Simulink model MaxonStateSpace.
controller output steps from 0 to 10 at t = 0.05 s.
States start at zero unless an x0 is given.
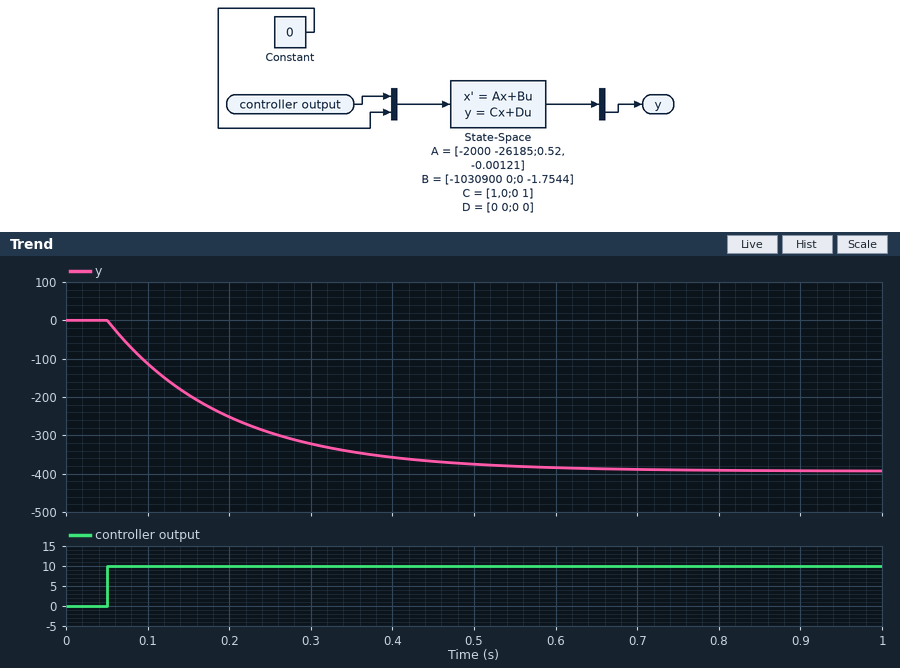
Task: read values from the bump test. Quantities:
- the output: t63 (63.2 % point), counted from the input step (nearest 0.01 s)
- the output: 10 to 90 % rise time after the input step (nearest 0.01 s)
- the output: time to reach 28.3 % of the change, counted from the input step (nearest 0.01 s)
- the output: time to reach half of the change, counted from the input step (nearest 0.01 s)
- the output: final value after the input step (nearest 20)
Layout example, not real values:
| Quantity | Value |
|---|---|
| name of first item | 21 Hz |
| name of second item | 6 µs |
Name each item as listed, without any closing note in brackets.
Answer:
| Quantity | Value |
|---|---|
| the output: t63 (63.2 % point), counted from the input step | 0.15 s |
| the output: 10 to 90 % rise time after the input step | 0.32 s |
| the output: time to reach 28.3 % of the change, counted from the input step | 0.05 s |
| the output: time to reach half of the change, counted from the input step | 0.10 s |
| the output: final value after the input step | -400 |
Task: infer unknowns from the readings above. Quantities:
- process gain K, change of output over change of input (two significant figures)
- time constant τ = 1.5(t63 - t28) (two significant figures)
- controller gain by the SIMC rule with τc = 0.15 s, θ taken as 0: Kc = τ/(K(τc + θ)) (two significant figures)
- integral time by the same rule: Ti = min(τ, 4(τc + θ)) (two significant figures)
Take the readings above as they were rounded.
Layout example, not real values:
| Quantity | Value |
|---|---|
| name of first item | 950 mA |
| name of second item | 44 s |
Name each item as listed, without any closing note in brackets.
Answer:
| Quantity | Value |
|---|---|
| process gain K, change of output over change of input | -40 |
| time constant τ = 1.5(t63 - t28) | 0.15 s |
| controller gain by the SIMC rule with τc = 0.15 s, θ taken as 0: Kc = τ/(K(τc + θ)) | -0.025 |
| integral time by the same rule: Ti = min(τ, 4(τc + θ)) | 0.15 s |
